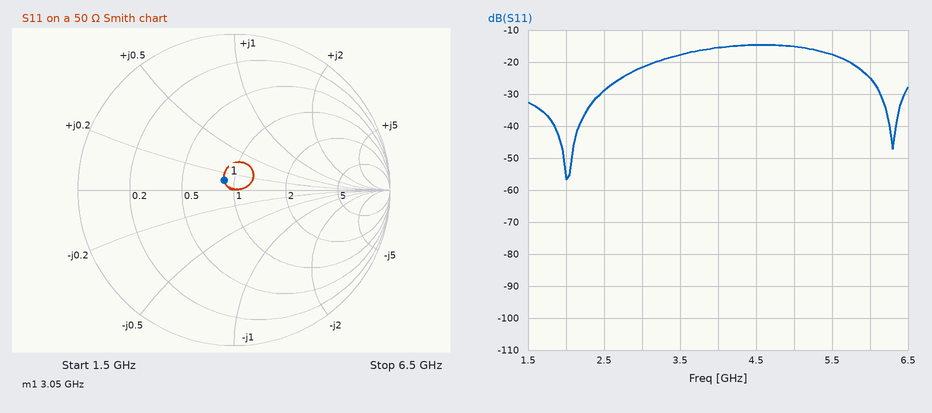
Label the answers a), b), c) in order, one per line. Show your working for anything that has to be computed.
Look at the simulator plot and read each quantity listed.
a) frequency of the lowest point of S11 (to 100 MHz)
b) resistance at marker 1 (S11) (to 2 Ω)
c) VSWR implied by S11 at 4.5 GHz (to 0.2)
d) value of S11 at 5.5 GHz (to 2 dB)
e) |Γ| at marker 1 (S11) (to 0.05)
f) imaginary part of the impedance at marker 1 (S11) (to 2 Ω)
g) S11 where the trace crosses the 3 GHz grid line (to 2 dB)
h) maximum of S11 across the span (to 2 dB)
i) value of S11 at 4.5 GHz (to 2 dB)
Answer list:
a) 2.0 GHz
b) 44 Ω
c) |Γ| = 10^(-14/20) = 0.1995; VSWR = (1 + 0.1995)/(1 − 0.1995) ≈ 1.50, so 1.4 to the nearest 0.2
d) -18 dB
e) 0.10
f) +6 Ω
g) -22 dB
h) -14 dB
i) -14 dB
